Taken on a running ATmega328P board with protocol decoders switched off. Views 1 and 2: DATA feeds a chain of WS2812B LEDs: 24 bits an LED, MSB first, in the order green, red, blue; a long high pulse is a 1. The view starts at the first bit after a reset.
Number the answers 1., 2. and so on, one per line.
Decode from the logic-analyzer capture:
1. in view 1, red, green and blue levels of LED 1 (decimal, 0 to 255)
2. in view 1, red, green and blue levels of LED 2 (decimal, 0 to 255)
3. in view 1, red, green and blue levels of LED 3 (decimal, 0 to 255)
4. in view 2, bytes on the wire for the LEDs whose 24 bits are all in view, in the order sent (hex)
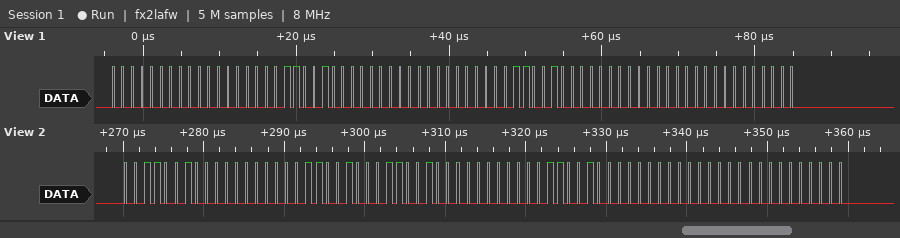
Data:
1. 0, 0, 50
2. 0, 0, 50
3. 0, 0, 0
4. 32 00 32 32 00 32 00 00 00
